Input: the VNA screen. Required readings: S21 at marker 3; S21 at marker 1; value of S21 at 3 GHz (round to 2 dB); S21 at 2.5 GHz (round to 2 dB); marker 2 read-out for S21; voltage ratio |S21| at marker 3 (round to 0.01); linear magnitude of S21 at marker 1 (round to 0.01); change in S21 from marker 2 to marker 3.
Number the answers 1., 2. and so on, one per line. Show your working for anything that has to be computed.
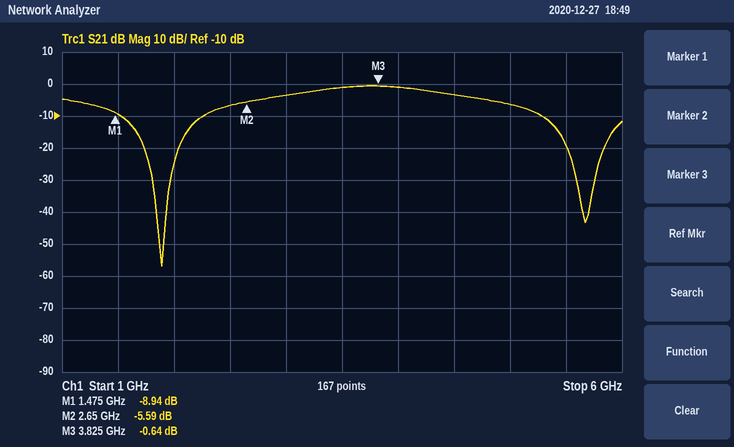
1. -0.64 dB
2. -8.94 dB
3. -4 dB
4. -6 dB
5. -5.59 dB
6. 10^(-0.64/20) ≈ 0.93
7. 10^(-8.94/20) ≈ 0.36
8. -0.64 − (-5.59) = 4.95 dB
